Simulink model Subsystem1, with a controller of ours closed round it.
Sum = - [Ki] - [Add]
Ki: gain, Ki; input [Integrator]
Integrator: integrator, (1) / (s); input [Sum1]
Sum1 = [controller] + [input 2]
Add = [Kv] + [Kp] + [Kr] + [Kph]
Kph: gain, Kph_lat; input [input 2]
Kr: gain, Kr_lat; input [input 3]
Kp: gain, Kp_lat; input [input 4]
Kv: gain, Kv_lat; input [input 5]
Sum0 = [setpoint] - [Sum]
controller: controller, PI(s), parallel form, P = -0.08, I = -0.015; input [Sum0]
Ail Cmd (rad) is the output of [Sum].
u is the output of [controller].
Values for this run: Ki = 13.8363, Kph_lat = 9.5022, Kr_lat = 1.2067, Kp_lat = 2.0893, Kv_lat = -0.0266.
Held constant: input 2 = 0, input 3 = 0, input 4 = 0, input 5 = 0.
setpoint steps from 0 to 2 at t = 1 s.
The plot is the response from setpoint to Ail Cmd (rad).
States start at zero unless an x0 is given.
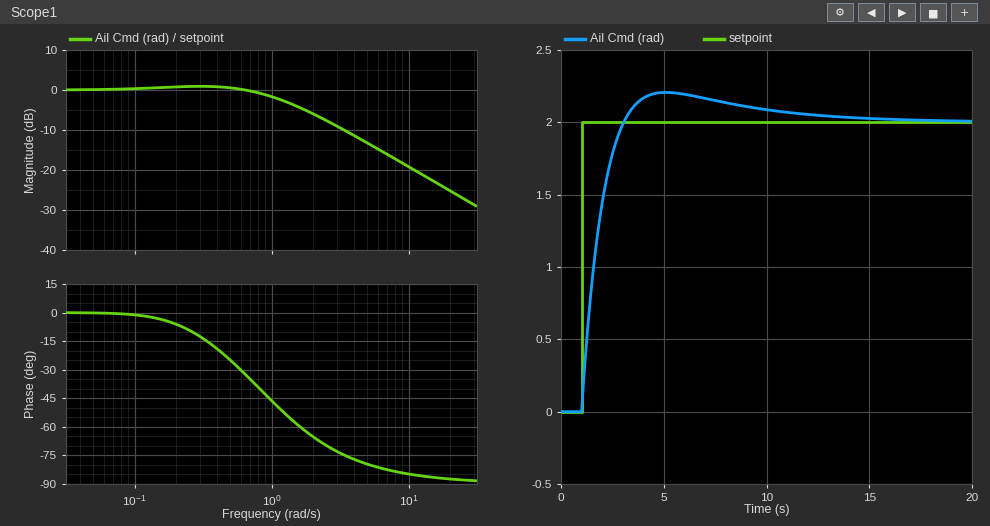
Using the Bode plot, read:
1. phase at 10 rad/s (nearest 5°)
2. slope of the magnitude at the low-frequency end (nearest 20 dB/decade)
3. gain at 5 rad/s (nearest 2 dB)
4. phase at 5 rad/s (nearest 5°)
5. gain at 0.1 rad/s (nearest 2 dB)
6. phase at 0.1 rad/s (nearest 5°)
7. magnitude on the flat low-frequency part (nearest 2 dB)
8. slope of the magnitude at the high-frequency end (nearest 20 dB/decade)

-85°
0 dB/decade
-14 dB
-80°
0 dB
0°
0 dB
-20 dB/decade
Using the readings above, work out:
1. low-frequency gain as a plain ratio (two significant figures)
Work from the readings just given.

1.0
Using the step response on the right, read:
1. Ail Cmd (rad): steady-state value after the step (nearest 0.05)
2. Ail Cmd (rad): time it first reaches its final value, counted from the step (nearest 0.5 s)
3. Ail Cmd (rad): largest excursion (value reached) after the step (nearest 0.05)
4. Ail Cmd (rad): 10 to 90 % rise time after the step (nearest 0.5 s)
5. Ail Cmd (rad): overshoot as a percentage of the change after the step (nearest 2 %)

2.00
2.0 s
2.20
1.5 s
10 %
